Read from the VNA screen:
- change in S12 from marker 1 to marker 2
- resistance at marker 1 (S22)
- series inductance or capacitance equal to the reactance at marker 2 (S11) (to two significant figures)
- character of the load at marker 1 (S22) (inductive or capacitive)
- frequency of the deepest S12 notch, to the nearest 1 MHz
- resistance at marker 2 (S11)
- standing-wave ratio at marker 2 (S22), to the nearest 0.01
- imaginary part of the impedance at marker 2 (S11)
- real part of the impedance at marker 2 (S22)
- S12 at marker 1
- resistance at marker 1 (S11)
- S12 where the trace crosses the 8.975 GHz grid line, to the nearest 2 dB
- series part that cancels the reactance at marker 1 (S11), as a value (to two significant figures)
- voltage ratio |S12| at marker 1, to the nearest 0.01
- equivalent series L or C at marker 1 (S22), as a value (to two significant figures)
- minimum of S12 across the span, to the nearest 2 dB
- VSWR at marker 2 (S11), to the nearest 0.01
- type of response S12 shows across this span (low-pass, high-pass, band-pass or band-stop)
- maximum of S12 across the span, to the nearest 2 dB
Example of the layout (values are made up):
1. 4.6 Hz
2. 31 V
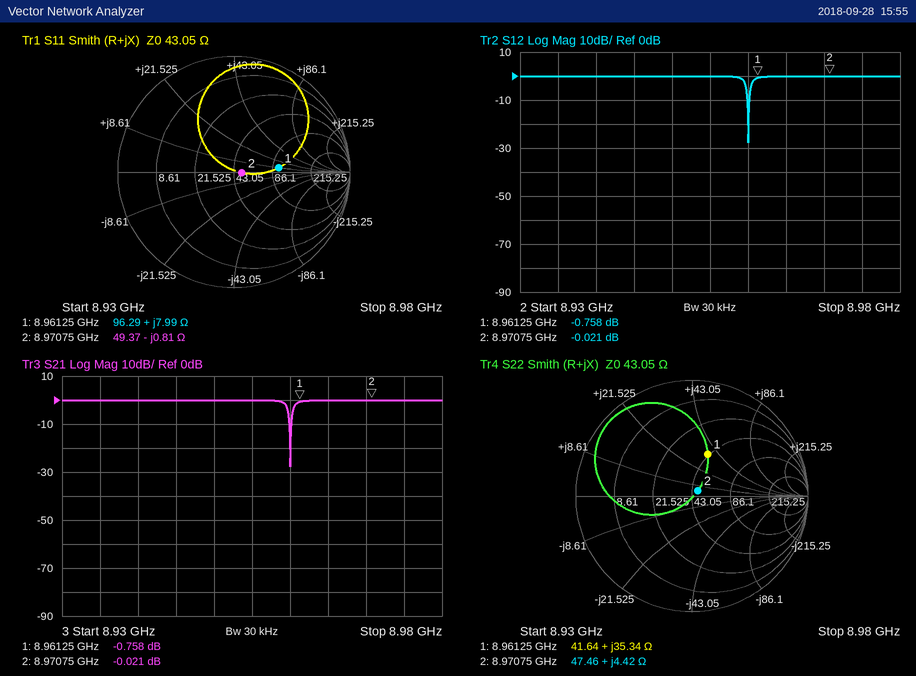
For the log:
1. 0.737 dB
2. 41.64 Ω
3. 22 pF
4. inductive
5. 8.960 GHz
6. 49.37 Ω
7. 1.15
8. -0.81 Ω
9. 47.46 Ω
10. -0.758 dB
11. 96.29 Ω
12. 0 dB
13. 2.2 pF
14. 0.92
15. 630 pH
16. -28 dB
17. 1.15
18. band-stop
19. 0 dB
